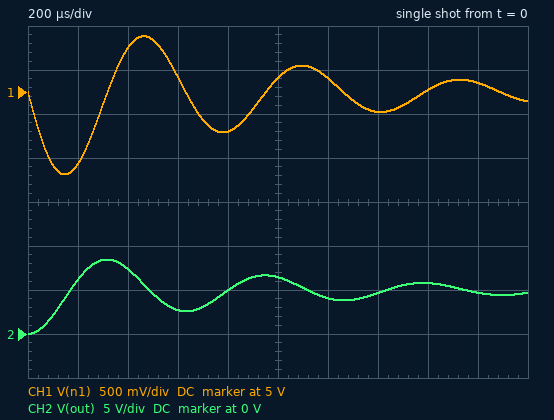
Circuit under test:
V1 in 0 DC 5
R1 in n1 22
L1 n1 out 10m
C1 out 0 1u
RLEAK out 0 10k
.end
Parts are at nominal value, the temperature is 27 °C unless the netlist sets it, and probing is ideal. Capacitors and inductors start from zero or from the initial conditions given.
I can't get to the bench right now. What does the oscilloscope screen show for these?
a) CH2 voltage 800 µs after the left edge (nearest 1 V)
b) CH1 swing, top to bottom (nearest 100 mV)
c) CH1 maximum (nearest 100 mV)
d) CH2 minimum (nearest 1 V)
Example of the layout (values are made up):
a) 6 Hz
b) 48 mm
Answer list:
a) 5 V
b) 1.6 V
c) 5.6 V
d) 0 V
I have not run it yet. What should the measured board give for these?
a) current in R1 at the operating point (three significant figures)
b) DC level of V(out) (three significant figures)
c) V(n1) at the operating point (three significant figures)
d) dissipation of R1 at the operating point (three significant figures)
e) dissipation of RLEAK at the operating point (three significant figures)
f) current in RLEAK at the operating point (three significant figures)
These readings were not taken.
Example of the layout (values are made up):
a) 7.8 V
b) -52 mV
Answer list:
a) 499 µA
b) 4.99 V
c) 4.99 V
d) 5.48 µW
e) 2.49 mW
f) 499 µA
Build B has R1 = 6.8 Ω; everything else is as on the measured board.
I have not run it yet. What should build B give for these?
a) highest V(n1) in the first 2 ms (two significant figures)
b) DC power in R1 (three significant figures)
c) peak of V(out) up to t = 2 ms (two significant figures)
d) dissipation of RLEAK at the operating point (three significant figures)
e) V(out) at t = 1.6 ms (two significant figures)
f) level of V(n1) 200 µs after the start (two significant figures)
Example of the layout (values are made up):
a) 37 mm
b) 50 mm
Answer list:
a) 5.3 V
b) 1.70 µW
c) 9.4 V
d) 2.50 mW
e) 7.6 V
f) 4.7 V
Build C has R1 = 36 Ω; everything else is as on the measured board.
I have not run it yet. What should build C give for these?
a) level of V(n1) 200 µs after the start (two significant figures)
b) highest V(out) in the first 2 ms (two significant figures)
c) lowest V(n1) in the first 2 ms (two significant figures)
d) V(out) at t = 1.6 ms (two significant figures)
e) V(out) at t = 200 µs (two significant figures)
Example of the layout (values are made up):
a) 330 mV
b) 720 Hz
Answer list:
a) 3.8 V
b) 7.7 V
c) 3.6 V
d) 5.2 V
e) 5.7 V
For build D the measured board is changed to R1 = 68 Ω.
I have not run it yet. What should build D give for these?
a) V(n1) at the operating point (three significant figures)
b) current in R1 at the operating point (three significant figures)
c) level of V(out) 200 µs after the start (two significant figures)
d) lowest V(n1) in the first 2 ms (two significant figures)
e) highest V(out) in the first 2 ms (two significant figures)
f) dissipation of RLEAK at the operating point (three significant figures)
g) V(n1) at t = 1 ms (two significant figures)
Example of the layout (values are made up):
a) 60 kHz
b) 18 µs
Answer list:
a) 4.97 V
b) 497 µA
c) 4.9 V
d) 2.8 V
e) 6.5 V
f) 2.47 mW
g) 5.0 V
